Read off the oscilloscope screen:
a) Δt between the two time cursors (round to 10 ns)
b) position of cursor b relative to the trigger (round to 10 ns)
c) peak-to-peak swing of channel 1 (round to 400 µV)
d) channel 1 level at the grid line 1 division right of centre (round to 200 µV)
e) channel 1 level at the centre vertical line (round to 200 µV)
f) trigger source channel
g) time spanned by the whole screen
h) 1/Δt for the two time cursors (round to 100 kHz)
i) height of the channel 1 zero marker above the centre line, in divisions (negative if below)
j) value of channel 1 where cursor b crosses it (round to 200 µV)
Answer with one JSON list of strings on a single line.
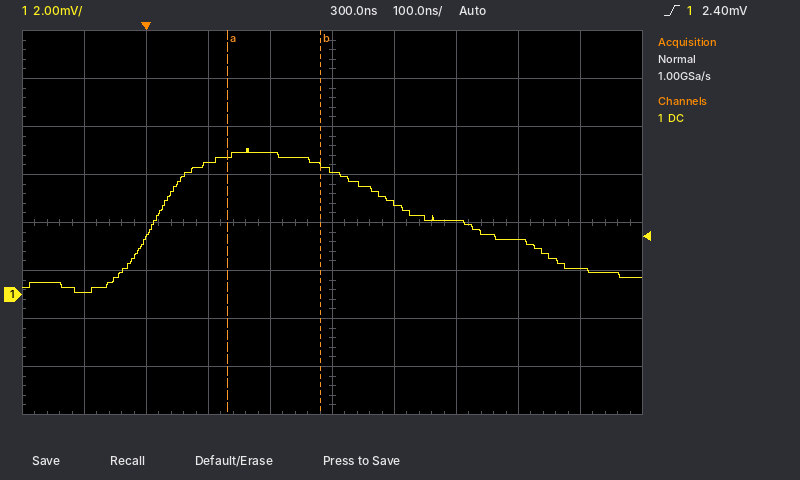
["150 ns", "+280 ns", "6.0 mV", "3.8 mV", "5.2 mV", "channel 1", "1 µs", "6.7 MHz", "-1.5 div", "5.4 mV"]
